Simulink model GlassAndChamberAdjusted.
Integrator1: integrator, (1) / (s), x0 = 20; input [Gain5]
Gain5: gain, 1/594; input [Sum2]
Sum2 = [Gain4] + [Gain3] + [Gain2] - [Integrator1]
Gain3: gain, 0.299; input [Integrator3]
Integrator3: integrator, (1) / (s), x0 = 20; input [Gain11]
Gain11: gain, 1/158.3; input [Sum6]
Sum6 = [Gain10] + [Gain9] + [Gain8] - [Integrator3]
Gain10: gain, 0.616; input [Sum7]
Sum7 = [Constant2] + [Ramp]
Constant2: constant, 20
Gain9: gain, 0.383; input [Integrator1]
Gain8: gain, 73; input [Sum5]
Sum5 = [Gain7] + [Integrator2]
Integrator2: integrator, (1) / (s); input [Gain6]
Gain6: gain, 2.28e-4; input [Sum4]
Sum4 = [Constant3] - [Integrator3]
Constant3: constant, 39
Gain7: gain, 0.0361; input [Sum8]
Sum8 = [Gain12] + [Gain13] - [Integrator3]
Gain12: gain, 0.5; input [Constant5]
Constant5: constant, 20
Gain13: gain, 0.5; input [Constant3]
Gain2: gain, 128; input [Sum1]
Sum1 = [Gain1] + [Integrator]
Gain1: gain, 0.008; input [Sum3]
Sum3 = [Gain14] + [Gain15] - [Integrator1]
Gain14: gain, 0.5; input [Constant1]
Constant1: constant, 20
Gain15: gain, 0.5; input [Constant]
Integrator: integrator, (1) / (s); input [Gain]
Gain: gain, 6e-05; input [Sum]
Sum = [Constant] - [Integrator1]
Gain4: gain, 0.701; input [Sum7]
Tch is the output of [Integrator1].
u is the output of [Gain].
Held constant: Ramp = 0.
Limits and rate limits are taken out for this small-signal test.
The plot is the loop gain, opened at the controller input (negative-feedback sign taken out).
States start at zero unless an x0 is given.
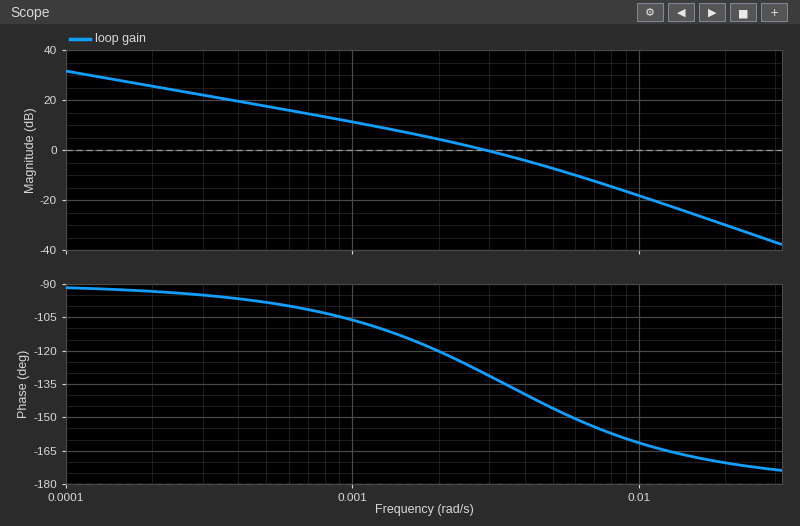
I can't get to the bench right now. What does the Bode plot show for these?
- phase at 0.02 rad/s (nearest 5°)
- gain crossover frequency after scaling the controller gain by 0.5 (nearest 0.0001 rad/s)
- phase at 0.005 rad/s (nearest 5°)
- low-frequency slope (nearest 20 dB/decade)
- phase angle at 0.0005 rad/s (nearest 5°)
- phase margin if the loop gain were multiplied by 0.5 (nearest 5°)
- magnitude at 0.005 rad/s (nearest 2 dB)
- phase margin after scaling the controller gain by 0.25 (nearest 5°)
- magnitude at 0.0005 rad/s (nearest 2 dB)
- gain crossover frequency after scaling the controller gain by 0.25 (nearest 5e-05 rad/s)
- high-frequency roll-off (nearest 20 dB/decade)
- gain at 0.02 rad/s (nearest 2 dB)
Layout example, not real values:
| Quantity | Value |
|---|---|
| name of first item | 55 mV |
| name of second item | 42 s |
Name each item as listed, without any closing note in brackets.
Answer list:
| Quantity | Value |
|---|---|
| phase at 0.02 rad/s | -170° |
| gain crossover frequency after scaling the controller gain by 0.5 | 0.0017 rad/s |
| phase at 0.005 rad/s | -145° |
| low-frequency slope | -20 dB/decade |
| phase angle at 0.0005 rad/s | -100° |
| phase margin if the loop gain were multiplied by 0.5 | 65° |
| magnitude at 0.005 rad/s | -8 dB |
| phase margin after scaling the controller gain by 0.25 | 75° |
| magnitude at 0.0005 rad/s | 18 dB |
| gain crossover frequency after scaling the controller gain by 0.25 | 0.00090 rad/s |
| high-frequency roll-off | -40 dB/decade |
| gain at 0.02 rad/s | -30 dB |
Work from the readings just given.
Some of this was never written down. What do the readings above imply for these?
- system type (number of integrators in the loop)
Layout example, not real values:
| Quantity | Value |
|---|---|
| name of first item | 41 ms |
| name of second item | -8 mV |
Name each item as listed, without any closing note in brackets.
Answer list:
| Quantity | Value |
|---|---|
| system type | 1 |
